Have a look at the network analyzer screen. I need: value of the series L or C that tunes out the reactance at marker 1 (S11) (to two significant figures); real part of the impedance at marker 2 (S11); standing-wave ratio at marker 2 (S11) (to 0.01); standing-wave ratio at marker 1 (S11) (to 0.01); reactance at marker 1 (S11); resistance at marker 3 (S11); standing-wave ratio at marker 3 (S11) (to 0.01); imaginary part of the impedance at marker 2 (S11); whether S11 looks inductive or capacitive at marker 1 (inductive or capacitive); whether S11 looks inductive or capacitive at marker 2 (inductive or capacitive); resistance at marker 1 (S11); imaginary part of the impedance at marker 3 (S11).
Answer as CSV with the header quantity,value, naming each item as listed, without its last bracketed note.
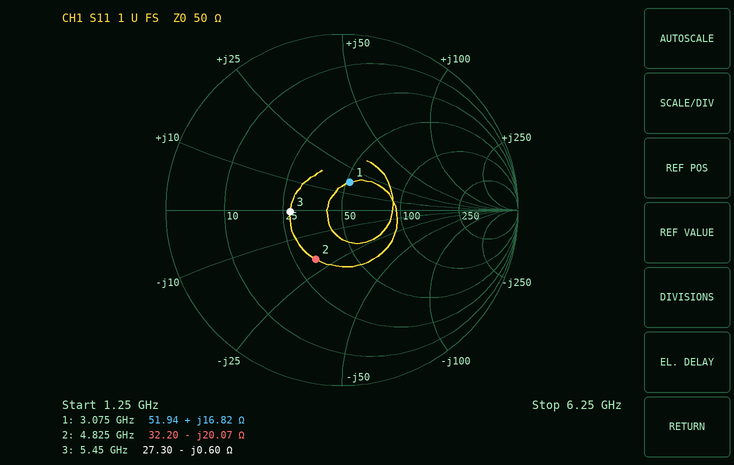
quantity,value
value of the series L or C that tunes out the reactance at marker 1 (S11),3.1 pF
real part of the impedance at marker 2,32.20 Ω
standing-wave ratio at marker 2 (S11),1.93
standing-wave ratio at marker 1 (S11),1.39
reactance at marker 1,+16.82 Ω
resistance at marker 3,27.30 Ω
standing-wave ratio at marker 3 (S11),1.83
imaginary part of the impedance at marker 2,-20.07 Ω
whether S11 looks inductive or capacitive at marker 1,inductive
whether S11 looks inductive or capacitive at marker 2,capacitive
resistance at marker 1,51.94 Ω
imaginary part of the impedance at marker 3,-0.60 Ω
